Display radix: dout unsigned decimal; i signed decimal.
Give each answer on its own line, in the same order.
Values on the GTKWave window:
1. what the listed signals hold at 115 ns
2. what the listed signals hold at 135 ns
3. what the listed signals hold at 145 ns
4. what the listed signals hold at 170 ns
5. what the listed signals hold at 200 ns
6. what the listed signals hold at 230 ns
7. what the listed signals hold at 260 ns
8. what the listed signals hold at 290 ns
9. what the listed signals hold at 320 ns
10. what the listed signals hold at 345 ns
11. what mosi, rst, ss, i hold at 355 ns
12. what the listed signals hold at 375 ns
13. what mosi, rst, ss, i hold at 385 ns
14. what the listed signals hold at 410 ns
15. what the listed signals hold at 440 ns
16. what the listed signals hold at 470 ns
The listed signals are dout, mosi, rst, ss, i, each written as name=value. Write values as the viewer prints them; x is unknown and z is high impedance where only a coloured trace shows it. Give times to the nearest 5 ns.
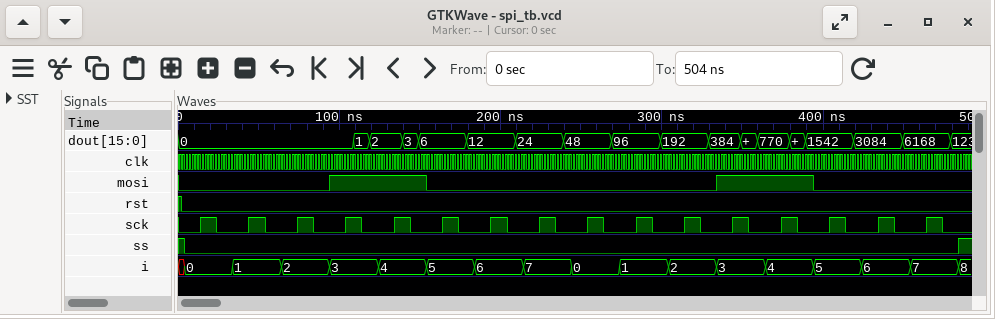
dout=1, mosi=1, rst=0, ss=0, i=3
dout=2, mosi=1, rst=0, ss=0, i=4
dout=3, mosi=1, rst=0, ss=0, i=4
dout=6, mosi=0, rst=0, ss=0, i=5
dout=12, mosi=0, rst=0, ss=0, i=6
dout=24, mosi=0, rst=0, ss=0, i=7
dout=48, mosi=0, rst=0, ss=0, i=0
dout=96, mosi=0, rst=0, ss=0, i=1
dout=192, mosi=0, rst=0, ss=0, i=2
dout=384, mosi=1, rst=0, ss=0, i=3
mosi=1, rst=0, ss=0, i=3
dout=770, mosi=1, rst=0, ss=0, i=4
mosi=1, rst=0, ss=0, i=4
dout=1542, mosi=0, rst=0, ss=0, i=5
dout=3084, mosi=0, rst=0, ss=0, i=6
dout=6168, mosi=0, rst=0, ss=0, i=7
